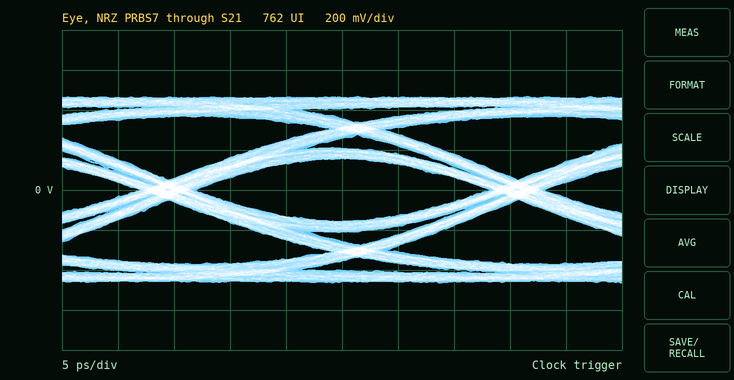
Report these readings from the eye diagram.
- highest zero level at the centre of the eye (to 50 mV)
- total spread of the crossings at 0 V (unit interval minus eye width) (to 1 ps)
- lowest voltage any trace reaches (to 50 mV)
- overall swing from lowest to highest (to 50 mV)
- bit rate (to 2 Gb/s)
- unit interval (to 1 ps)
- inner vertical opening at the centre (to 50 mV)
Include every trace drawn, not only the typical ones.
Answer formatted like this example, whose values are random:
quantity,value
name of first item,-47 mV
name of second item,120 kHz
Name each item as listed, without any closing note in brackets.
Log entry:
quantity,value
highest zero level at the centre of the eye,-150 mV
total spread of the crossings at 0 V (unit interval minus eye width),5 ps
lowest voltage any trace reaches,-450 mV
overall swing from lowest to highest,950 mV
bit rate,32 Gb/s
unit interval,31 ps
inner vertical opening at the centre,300 mV
